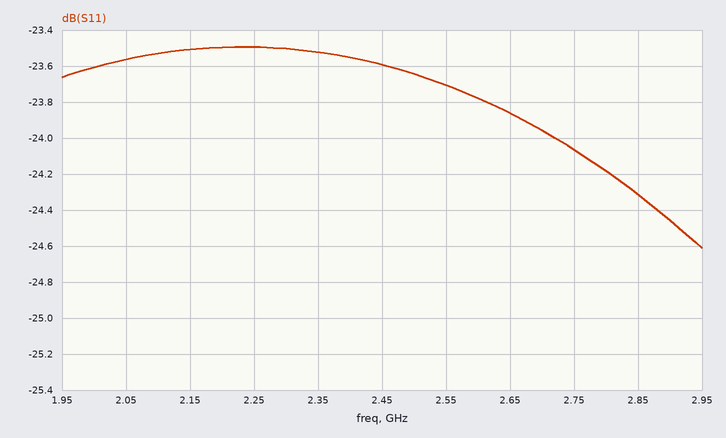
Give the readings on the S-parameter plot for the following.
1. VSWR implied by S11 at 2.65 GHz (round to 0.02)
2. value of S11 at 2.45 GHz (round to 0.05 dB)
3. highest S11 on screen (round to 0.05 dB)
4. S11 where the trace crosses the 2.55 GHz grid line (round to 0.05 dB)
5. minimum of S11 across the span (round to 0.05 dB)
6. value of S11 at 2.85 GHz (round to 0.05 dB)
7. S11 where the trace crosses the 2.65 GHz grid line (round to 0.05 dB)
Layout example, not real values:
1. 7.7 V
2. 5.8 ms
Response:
1. 1.14
2. -23.60 dB
3. -23.50 dB
4. -23.70 dB
5. -24.60 dB
6. -24.30 dB
7. -23.85 dB
